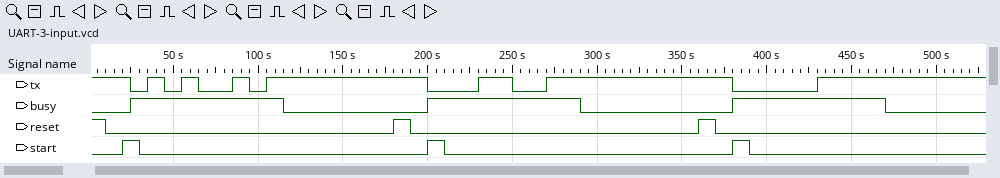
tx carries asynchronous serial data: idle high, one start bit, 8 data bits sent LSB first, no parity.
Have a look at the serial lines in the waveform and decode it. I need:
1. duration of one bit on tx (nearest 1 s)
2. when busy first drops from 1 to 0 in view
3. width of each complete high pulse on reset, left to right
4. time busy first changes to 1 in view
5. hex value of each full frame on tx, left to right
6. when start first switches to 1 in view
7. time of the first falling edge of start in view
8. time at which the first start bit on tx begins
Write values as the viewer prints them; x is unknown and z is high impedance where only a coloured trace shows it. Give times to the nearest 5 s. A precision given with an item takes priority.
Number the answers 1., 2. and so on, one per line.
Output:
1. 10 s
2. 115 s
3. 10 s, 10 s
4. 25 s
5. A5, CC, F0
6. 20 s
7. 30 s
8. 25 s
